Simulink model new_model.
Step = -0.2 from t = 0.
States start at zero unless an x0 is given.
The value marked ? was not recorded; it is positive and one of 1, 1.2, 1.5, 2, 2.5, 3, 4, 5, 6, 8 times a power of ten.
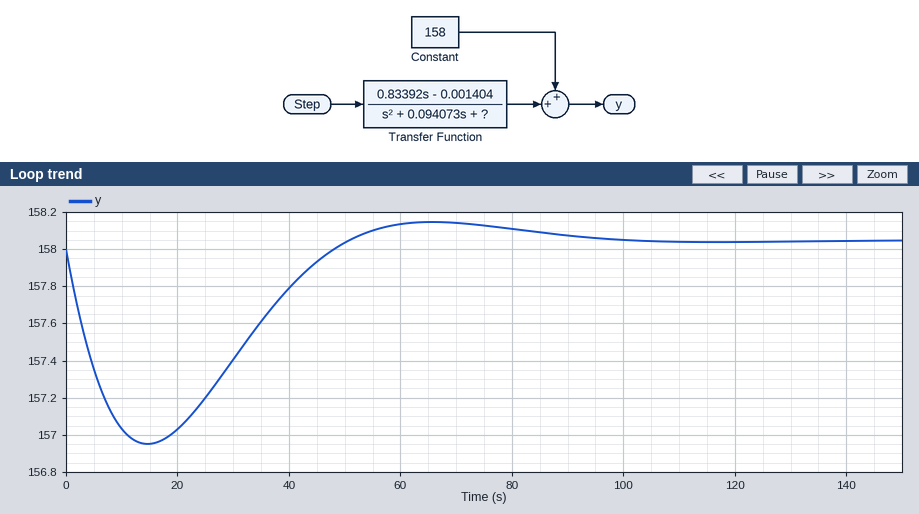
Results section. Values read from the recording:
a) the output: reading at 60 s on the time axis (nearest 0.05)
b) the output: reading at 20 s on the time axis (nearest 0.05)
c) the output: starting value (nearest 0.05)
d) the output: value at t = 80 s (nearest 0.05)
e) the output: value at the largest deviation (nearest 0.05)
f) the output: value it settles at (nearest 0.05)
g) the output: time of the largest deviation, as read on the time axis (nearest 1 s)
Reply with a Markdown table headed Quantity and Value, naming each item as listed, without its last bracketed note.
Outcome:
| Quantity | Value |
|---|---|
| the output: reading at 60 s on the time axis | 158.15 |
| the output: reading at 20 s on the time axis | 157.05 |
| the output: starting value | 158.00 |
| the output: value at t = 80 s | 158.10 |
| the output: value at the largest deviation | 156.95 |
| the output: value it settles at | 158.05 |
| the output: time of the largest deviation, as read on the time axis | 15 s |
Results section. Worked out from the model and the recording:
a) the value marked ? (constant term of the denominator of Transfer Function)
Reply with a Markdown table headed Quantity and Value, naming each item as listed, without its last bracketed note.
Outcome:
| Quantity | Value |
|---|---|
| the value marked ? | 0.006 |
